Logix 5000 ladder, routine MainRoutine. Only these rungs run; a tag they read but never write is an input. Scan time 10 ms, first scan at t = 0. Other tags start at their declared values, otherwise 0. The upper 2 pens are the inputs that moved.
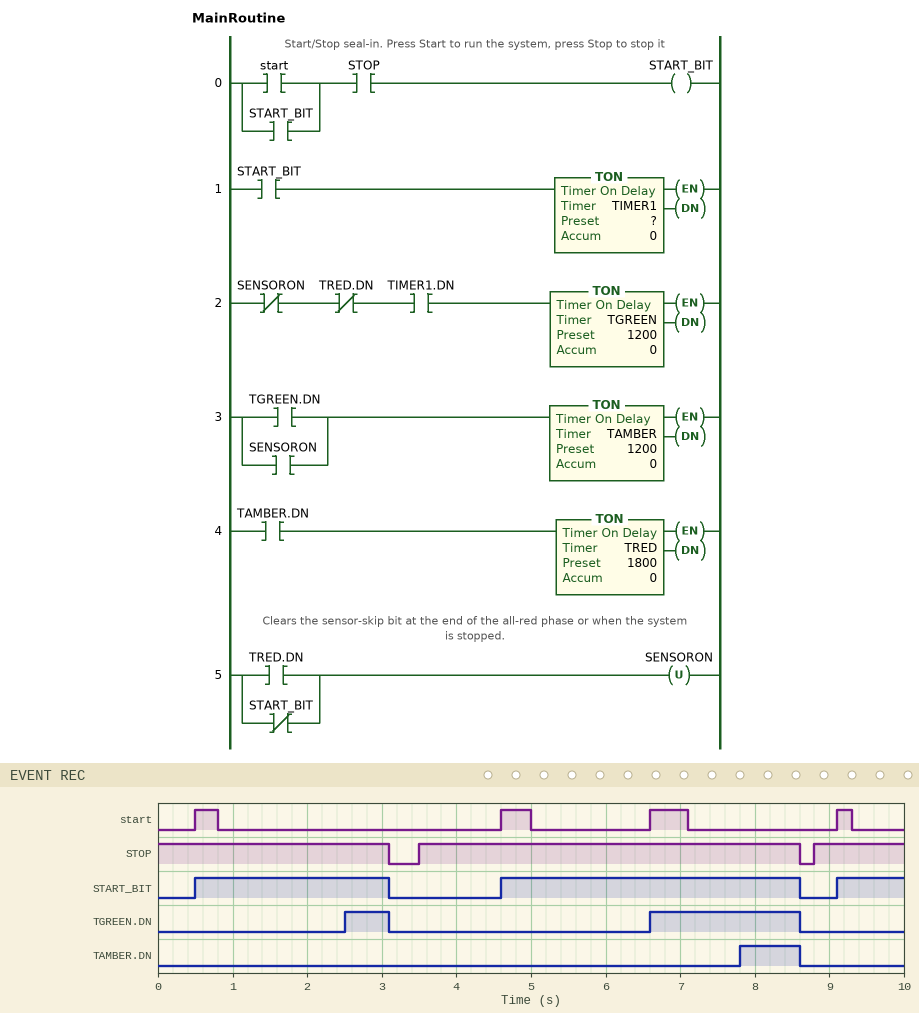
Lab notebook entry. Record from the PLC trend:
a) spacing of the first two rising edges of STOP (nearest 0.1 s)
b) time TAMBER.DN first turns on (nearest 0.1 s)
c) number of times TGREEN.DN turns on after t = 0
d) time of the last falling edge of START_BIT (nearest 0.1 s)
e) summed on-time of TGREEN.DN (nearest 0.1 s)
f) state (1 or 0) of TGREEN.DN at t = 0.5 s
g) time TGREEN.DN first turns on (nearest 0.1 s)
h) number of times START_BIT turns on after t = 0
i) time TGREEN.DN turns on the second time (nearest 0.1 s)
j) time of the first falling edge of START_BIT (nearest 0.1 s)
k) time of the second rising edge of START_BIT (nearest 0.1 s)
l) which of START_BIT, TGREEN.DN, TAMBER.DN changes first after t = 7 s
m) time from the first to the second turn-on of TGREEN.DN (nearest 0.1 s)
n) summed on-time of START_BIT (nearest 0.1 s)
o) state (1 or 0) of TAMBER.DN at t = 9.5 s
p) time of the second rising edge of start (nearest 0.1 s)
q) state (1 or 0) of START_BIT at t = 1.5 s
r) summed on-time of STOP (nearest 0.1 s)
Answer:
5.3 s
7.8 s
2
8.6 s
2.6 s
0
2.5 s
3
6.6 s
3.1 s
4.6 s
TAMBER.DN
4.1 s
7.5 s
0
4.6 s
1
9.4 s
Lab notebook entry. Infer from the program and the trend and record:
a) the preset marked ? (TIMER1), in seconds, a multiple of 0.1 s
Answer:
0.8 s
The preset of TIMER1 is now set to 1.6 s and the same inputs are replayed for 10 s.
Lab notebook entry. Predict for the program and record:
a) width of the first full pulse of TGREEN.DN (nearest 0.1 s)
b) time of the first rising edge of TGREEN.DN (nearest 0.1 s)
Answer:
1.2 s
7.4 s
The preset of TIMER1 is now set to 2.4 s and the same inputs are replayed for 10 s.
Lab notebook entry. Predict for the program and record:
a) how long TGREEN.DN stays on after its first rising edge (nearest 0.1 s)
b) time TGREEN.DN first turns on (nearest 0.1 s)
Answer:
0.4 s
8.2 s
